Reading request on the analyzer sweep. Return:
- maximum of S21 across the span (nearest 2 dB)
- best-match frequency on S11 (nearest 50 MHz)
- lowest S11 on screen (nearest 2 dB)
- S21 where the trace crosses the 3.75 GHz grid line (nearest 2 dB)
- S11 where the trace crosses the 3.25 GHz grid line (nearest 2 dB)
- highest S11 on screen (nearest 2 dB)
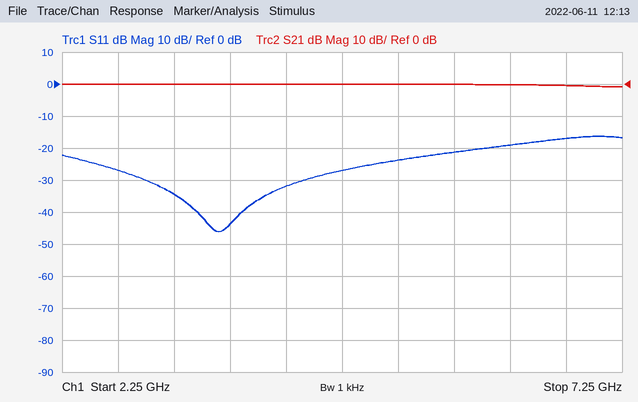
0 dB
3.65 GHz
-46 dB
0 dB
-34 dB
-16 dB
